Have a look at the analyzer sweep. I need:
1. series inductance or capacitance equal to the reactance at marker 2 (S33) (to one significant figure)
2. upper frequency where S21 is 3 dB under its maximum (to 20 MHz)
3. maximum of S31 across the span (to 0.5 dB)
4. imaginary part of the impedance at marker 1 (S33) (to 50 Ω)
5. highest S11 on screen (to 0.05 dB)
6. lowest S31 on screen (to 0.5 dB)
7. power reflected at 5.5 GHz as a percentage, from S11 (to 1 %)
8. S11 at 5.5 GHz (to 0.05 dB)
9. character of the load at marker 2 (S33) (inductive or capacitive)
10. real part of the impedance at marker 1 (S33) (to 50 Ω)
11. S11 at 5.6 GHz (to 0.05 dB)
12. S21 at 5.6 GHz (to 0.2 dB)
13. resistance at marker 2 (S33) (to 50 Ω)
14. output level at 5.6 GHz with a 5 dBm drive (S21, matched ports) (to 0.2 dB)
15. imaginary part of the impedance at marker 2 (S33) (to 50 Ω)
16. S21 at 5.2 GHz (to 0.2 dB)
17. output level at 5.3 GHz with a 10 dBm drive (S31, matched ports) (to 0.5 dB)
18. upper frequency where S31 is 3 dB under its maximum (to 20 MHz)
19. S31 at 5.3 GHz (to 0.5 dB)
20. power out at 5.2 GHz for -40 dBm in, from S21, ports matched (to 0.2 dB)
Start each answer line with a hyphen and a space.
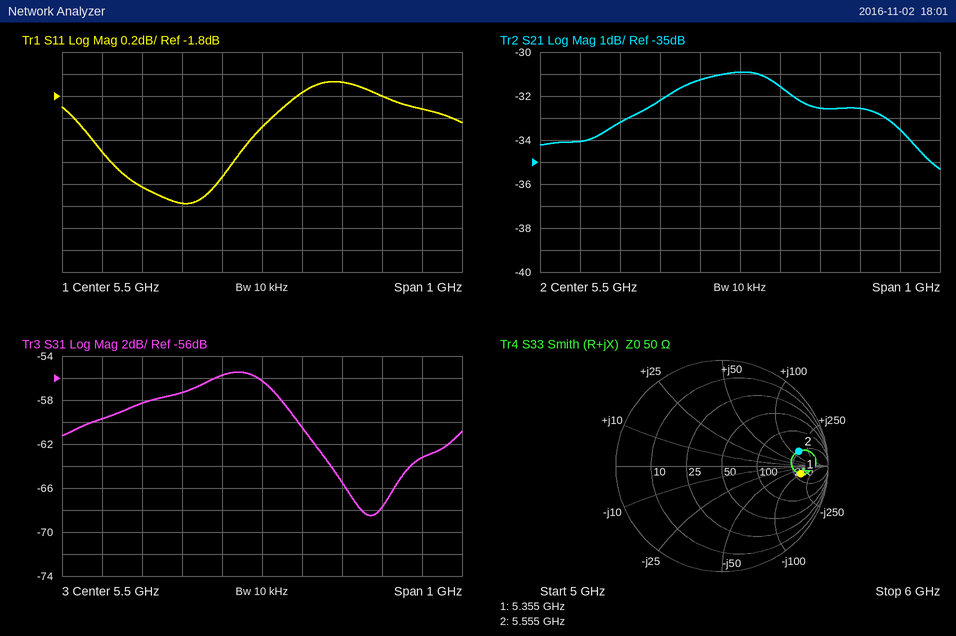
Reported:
- 4 nH
- 5.92 GHz
- -55.5 dB
- -100 Ω
- -1.65 dB
- -68.5 dB
- 62 %
- -2.10 dB
- inductive
- 300 Ω
- -1.75 dB
- -31.6 dB
- 250 Ω
- -26.6 dBm
- +150 Ω
- -33.2 dB
- -47.5 dBm
- 5.56 GHz
- -57.5 dB
- -73.2 dBm
